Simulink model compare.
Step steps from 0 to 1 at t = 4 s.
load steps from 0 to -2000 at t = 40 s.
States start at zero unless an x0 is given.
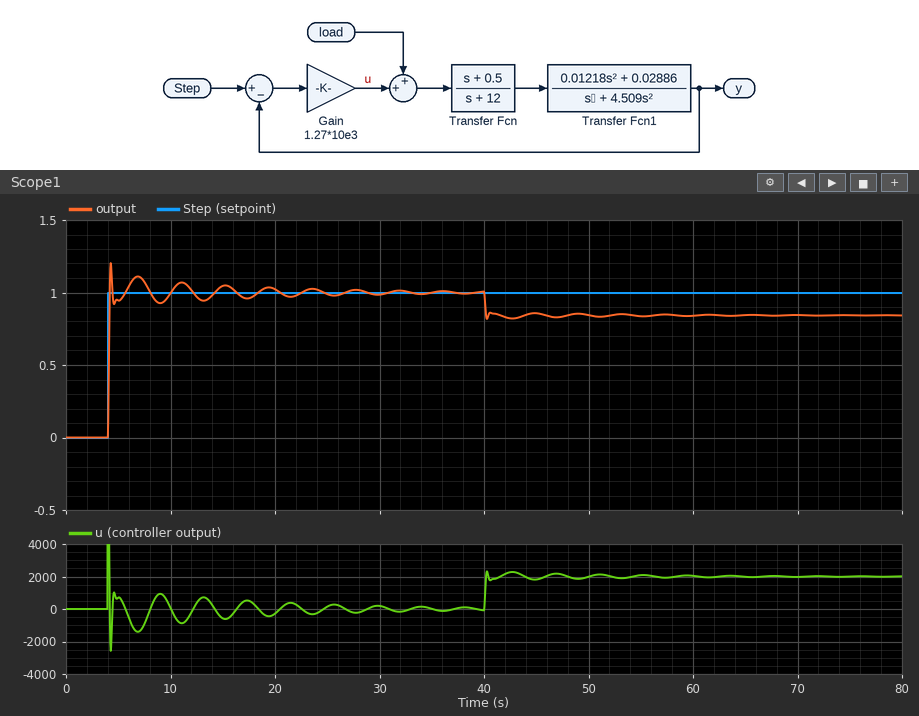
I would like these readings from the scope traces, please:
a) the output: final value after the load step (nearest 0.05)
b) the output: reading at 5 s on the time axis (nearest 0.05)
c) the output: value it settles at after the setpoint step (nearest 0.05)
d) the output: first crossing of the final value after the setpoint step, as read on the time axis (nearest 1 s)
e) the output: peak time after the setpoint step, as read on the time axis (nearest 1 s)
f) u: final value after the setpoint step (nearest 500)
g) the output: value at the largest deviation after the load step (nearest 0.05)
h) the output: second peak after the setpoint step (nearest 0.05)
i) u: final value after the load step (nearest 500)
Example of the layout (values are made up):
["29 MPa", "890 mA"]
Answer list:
["0.85", "0.95", "1.00", "4 s", "4 s", "0", "0.80", "1.10", "2000"]
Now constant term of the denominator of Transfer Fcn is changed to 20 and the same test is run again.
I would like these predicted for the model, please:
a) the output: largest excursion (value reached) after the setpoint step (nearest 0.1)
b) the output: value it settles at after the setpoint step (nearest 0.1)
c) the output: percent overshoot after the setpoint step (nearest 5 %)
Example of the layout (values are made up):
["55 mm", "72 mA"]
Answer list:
["1.2", "1.0", "15 %"]
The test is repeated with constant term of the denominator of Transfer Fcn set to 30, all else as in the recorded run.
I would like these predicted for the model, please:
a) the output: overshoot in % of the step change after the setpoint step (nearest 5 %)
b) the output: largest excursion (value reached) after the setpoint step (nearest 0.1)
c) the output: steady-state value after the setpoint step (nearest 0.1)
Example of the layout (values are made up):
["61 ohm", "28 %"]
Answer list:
["25 %", "1.2", "1.0"]
